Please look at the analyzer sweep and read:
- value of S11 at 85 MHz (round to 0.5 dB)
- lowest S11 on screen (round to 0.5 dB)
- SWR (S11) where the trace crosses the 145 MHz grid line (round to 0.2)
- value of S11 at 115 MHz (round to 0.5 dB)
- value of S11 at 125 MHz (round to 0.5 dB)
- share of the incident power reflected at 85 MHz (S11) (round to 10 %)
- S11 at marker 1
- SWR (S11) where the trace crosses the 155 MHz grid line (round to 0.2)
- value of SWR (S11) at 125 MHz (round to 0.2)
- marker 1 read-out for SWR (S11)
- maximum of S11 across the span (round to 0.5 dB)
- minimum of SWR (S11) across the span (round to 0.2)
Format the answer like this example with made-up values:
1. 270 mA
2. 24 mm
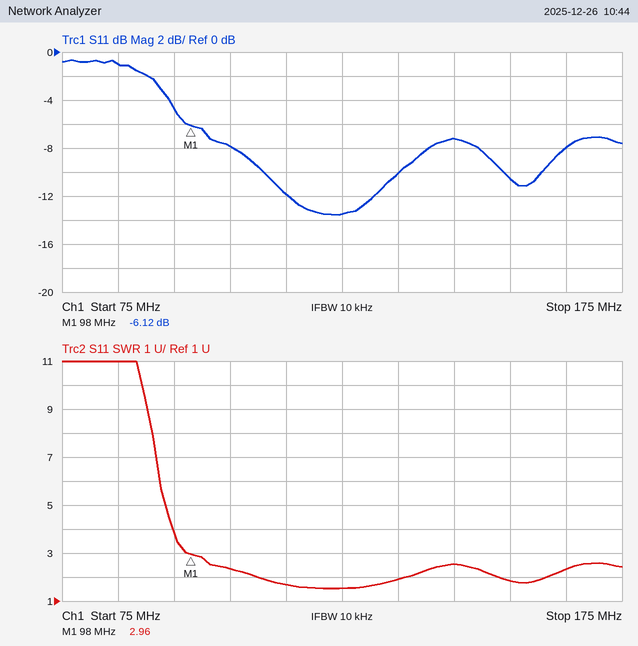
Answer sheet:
1. -1.0 dB
2. -13.5 dB
3. 2.6
4. -12.0 dB
5. -13.5 dB
6. 80 %
7. -6.12 dB
8. 1.8
9. 1.6
10. 2.96
11. -0.5 dB
12. 1.6
